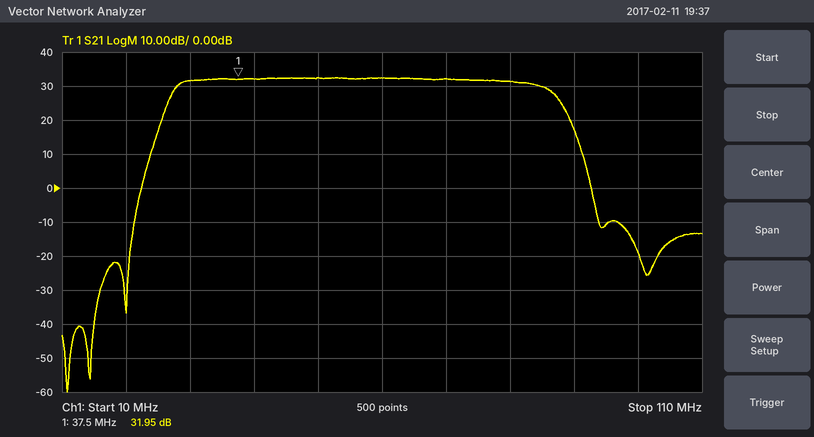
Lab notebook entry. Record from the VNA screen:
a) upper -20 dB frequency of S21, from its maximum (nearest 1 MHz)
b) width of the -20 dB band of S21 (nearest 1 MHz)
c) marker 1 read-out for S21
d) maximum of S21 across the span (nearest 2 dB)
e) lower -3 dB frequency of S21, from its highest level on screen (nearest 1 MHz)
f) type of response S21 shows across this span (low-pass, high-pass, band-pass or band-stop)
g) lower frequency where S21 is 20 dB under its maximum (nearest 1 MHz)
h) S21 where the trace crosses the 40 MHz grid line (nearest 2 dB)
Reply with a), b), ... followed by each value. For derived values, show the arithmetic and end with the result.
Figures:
a) 91 MHz
b) 91 MHz − 24 MHz = 67 MHz
c) 31.95 dB
d) 32 dB
e) 28 MHz
f) band-pass
g) 24 MHz
h) 32 dB
